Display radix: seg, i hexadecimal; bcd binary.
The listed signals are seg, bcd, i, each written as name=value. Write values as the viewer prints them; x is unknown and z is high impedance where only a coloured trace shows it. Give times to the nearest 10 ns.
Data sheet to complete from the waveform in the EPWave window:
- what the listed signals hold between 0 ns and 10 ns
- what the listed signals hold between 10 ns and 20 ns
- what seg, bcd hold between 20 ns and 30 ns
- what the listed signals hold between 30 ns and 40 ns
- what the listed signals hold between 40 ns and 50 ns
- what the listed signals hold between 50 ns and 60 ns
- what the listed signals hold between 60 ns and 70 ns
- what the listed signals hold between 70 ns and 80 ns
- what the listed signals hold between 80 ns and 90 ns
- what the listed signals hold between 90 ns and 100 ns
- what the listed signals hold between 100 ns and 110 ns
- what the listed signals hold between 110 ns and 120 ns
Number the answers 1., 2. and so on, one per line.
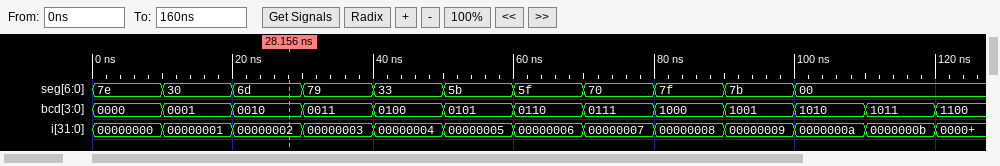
1. seg=7e, bcd=0000, i=00000000
2. seg=30, bcd=0001, i=00000001
3. seg=6d, bcd=0010
4. seg=79, bcd=0011, i=00000003
5. seg=33, bcd=0100, i=00000004
6. seg=5b, bcd=0101, i=00000005
7. seg=5f, bcd=0110, i=00000006
8. seg=70, bcd=0111, i=00000007
9. seg=7f, bcd=1000, i=00000008
10. seg=7b, bcd=1001, i=00000009
11. seg=00, bcd=1010, i=0000000a
12. seg=00, bcd=1011, i=0000000b
